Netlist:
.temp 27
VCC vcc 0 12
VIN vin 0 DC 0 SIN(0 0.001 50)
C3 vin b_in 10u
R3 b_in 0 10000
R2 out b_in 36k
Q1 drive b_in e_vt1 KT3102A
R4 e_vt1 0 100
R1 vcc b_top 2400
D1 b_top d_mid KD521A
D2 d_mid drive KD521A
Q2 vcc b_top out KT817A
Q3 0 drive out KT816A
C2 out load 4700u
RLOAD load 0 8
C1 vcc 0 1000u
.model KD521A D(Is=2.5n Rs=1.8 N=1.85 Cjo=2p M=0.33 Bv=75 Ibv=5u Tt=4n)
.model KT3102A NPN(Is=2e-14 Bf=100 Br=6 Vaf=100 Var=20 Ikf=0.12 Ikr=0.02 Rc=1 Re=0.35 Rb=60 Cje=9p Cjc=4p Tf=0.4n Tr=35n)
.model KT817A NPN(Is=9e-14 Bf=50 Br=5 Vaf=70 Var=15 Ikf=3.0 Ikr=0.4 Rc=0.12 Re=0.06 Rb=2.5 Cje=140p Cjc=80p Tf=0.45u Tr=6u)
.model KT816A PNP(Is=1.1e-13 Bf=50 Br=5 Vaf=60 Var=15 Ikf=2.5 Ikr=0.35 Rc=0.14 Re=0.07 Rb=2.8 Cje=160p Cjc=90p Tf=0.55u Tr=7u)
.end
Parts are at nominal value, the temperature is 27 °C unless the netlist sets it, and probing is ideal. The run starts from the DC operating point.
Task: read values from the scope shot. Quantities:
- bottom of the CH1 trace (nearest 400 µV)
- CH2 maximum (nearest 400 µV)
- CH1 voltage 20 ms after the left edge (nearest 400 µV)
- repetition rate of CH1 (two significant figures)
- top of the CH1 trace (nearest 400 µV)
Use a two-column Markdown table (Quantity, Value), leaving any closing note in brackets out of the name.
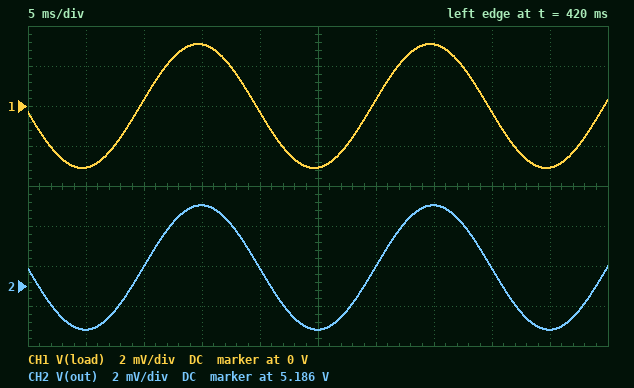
| Quantity | Value |
|---|---|
| bottom of the CH1 trace | -3.2 mV |
| CH2 maximum | 5.1900 V |
| CH1 voltage 20 ms after the left edge | -400 µV |
| repetition rate of CH1 | 50 Hz |
| top of the CH1 trace | 3.2 mV |
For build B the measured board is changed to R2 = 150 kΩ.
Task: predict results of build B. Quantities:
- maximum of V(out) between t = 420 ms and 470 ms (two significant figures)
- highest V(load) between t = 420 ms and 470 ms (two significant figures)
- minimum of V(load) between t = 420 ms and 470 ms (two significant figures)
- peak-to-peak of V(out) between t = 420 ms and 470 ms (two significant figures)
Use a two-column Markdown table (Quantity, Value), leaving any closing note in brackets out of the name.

| Quantity | Value |
|---|---|
| maximum of V(out) between t = 420 ms and 470 ms | 11 V |
| highest V(load) between t = 420 ms and 470 ms | 1.1 mV |
| minimum of V(load) between t = 420 ms and 470 ms | -1.1 mV |
| peak-to-peak of V(out) between t = 420 ms and 470 ms | 2.3 mV |
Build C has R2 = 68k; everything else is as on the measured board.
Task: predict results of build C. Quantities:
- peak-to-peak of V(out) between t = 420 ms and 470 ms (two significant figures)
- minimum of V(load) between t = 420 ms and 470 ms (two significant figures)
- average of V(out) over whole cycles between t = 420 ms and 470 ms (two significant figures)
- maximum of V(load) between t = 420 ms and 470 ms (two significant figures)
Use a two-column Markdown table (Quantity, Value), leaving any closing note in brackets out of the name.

| Quantity | Value |
|---|---|
| peak-to-peak of V(out) between t = 420 ms and 470 ms | 5.9 mV |
| minimum of V(load) between t = 420 ms and 470 ms | -2.9 mV |
| average of V(out) over whole cycles between t = 420 ms and 470 ms | 7.4 V |
| maximum of V(load) between t = 420 ms and 470 ms | 2.9 mV |
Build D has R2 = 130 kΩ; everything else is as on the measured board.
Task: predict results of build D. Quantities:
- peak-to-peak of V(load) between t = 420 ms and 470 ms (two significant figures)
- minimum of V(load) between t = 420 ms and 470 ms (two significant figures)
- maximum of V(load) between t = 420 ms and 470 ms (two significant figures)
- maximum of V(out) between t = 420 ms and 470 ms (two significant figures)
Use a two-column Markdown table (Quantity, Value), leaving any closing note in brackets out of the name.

| Quantity | Value |
|---|---|
| peak-to-peak of V(load) between t = 420 ms and 470 ms | 3.7 mV |
| minimum of V(load) between t = 420 ms and 470 ms | -1.9 mV |
| maximum of V(load) between t = 420 ms and 470 ms | 1.9 mV |
| maximum of V(out) between t = 420 ms and 470 ms | 10 V |
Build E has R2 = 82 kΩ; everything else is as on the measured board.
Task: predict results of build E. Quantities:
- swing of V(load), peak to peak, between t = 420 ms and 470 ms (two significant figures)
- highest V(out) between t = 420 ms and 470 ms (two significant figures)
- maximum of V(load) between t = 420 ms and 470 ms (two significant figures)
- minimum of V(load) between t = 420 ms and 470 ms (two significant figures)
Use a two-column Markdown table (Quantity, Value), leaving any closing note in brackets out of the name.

| Quantity | Value |
|---|---|
| swing of V(load), peak to peak, between t = 420 ms and 470 ms | 5.6 mV |
| highest V(out) between t = 420 ms and 470 ms | 8.2 V |
| maximum of V(load) between t = 420 ms and 470 ms | 2.8 mV |
| minimum of V(load) between t = 420 ms and 470 ms | -2.8 mV |
